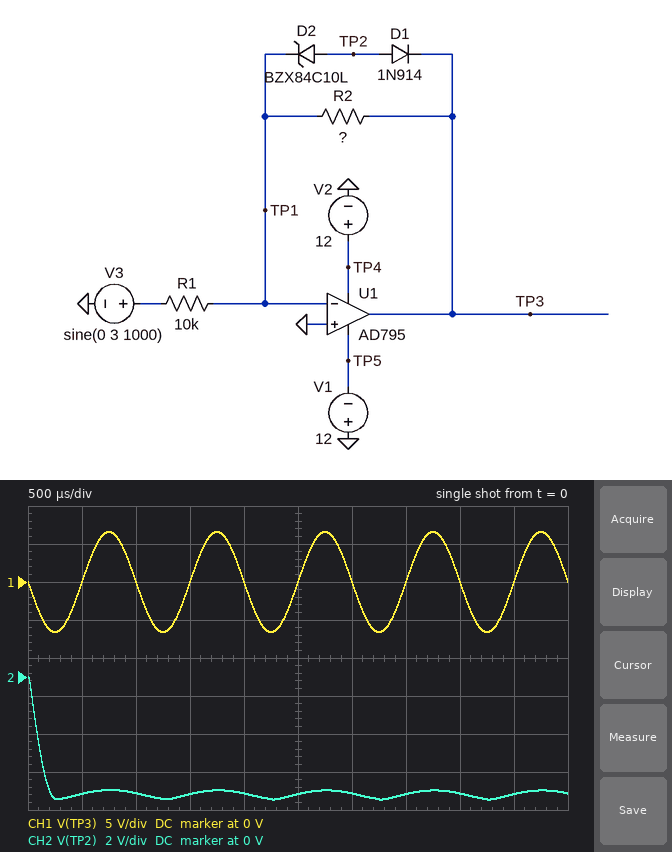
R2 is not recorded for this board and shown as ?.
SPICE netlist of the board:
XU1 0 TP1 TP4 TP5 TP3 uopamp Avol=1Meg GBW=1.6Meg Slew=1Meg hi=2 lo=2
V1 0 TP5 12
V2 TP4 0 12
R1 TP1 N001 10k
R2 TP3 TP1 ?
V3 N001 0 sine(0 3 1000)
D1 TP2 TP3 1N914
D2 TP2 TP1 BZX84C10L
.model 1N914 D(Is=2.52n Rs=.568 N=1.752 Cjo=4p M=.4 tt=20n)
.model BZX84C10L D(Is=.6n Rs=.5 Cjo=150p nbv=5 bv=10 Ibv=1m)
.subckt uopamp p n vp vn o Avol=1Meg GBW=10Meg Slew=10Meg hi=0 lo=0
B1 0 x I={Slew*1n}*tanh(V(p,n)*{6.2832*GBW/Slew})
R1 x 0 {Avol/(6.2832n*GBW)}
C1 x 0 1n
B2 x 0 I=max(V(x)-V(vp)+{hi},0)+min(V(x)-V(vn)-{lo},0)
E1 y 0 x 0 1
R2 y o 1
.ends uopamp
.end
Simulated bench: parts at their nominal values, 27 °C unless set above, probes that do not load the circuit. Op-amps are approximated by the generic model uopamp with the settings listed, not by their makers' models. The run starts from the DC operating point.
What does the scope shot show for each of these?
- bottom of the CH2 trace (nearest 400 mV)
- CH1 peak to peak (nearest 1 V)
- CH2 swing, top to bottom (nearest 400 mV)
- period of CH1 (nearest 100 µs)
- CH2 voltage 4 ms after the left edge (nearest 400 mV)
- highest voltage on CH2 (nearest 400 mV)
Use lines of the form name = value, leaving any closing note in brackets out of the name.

bottom of the CH2 trace = -6.4 V
CH1 peak to peak = 13 V
CH2 swing, top to bottom = 6.4 V
period of CH1 = 1.0 ms
CH2 voltage 4 ms after the left edge = -6.0 V
highest voltage on CH2 = 0 V
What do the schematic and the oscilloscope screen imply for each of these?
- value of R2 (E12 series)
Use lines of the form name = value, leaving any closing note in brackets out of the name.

value of R2 = 22 kΩ
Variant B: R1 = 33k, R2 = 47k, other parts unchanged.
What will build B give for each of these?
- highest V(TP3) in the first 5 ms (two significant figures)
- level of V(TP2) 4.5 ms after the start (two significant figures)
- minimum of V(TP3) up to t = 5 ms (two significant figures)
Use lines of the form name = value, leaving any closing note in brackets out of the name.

highest V(TP3) in the first 5 ms = 4.3 V
level of V(TP2) 4.5 ms after the start = -4.0 V
minimum of V(TP3) up to t = 5 ms = -4.3 V
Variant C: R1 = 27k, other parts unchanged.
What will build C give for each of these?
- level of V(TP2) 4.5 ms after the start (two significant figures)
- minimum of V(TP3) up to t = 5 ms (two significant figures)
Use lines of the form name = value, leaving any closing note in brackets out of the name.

level of V(TP2) 4.5 ms after the start = -2.2 V
minimum of V(TP3) up to t = 5 ms = -2.4 V
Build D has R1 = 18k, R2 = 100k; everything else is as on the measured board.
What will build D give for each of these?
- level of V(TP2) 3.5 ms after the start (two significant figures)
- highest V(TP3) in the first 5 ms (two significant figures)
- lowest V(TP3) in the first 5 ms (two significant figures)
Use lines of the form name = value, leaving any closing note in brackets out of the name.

level of V(TP2) 3.5 ms after the start = -8.5 V
highest V(TP3) in the first 5 ms = 10 V
lowest V(TP3) in the first 5 ms = -10 V
